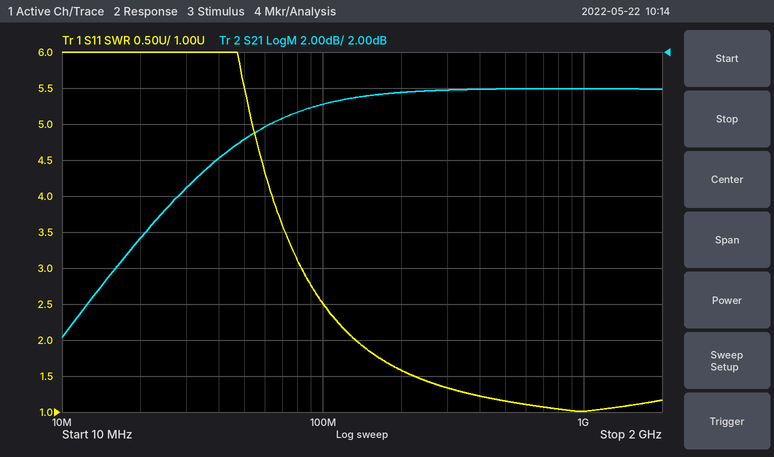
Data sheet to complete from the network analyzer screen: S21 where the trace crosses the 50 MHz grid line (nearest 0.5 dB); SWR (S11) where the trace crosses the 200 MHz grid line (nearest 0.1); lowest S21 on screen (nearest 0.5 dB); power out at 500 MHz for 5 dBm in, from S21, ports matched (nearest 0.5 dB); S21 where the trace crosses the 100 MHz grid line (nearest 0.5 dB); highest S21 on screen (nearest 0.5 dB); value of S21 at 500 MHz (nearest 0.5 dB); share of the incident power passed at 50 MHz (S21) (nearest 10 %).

-3.0 dB
1.6
-14.0 dB
5.0 dBm
-1.0 dB
0.0 dB
0.0 dB
50 %
